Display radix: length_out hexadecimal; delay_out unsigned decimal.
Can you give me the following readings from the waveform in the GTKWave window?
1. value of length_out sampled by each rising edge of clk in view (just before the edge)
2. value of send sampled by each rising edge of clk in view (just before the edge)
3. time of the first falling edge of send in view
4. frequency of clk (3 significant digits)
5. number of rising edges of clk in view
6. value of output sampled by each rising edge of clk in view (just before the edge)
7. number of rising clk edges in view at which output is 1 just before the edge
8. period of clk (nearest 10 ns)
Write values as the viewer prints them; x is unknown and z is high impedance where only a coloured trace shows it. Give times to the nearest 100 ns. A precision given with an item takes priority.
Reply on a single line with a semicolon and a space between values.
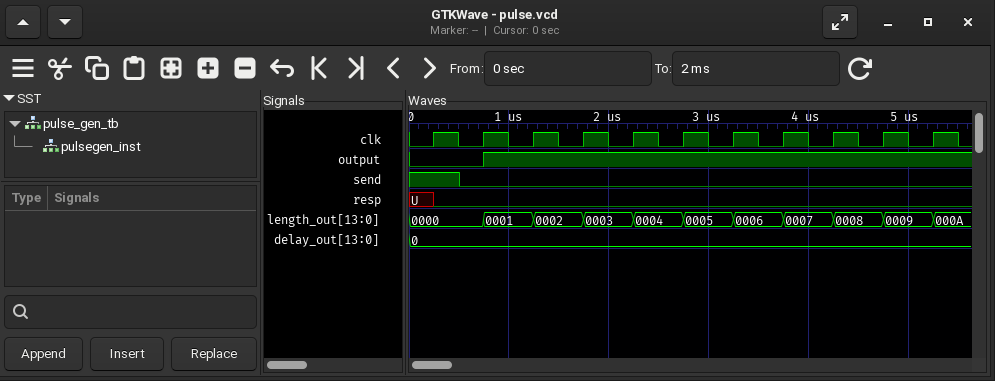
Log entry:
0000, 0000, 0001, 0002, 0003, 0004, 0005, 0006, 0007, 0008, 0009; 1 0 0 0 0 0 0 0 0 0 0; 500 ns; 2.00 MHz; 11; 0 0 1 1 1 1 1 1 1 1 1; 9; 500 ns
